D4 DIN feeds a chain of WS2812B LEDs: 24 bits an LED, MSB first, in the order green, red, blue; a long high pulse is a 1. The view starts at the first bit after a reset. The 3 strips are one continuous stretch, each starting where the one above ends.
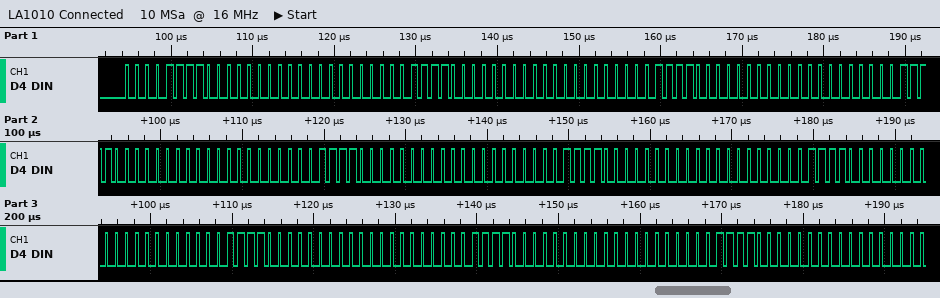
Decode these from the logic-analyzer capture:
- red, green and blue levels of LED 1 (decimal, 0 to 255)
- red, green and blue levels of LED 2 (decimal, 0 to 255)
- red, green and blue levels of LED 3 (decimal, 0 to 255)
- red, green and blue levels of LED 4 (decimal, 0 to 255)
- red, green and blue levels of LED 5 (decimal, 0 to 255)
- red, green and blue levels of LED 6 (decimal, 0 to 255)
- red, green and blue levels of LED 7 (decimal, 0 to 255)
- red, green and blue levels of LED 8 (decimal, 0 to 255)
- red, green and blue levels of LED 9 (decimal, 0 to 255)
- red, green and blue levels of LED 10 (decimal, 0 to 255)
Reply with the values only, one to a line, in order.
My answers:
0, 15, 0
0, 15, 0
0, 15, 0
0, 15, 0
0, 15, 0
0, 15, 0
0, 15, 0
0, 15, 0
0, 15, 0
0, 15, 0
